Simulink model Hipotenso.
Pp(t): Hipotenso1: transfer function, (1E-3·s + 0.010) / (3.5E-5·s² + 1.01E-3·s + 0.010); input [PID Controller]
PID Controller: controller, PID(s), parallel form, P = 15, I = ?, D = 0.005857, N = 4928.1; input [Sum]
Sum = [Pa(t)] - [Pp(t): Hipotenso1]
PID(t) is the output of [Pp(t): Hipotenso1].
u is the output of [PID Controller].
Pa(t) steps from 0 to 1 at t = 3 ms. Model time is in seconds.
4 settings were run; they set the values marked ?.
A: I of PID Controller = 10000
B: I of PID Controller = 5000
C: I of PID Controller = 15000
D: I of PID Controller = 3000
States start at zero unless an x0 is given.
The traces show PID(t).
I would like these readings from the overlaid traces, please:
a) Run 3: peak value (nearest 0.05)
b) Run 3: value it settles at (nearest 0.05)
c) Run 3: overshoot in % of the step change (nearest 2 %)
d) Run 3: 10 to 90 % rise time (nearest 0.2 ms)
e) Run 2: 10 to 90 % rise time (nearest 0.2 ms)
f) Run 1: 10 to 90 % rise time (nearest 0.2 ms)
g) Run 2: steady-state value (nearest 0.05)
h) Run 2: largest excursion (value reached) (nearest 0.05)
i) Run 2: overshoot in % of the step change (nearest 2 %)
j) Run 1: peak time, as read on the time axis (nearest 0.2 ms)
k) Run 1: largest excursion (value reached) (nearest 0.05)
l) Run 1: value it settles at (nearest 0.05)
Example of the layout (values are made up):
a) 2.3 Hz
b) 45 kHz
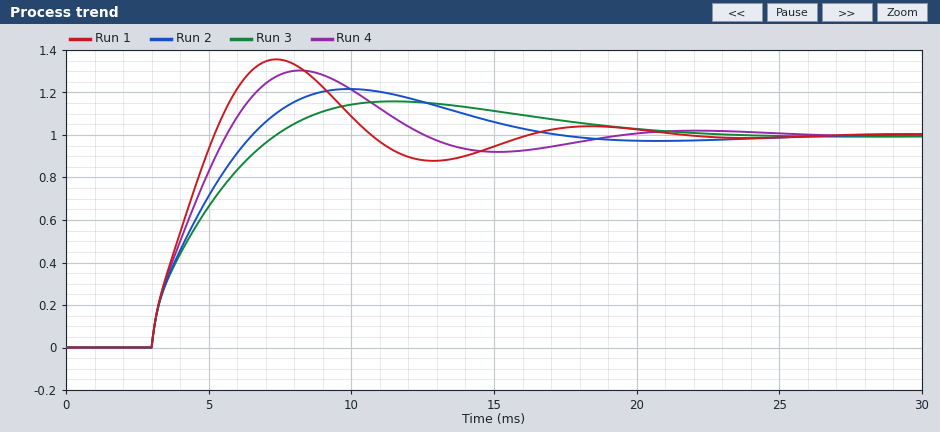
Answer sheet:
a) 1.15
b) 1.00
c) 16 %
d) 3.4 ms
e) 2.8 ms
f) 1.8 ms
g) 1.00
h) 1.20
i) 22 %
j) 7.4 ms
k) 1.35
l) 1.00
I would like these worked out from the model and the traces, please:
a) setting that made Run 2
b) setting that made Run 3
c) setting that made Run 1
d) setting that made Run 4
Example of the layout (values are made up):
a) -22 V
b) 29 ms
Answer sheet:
a) B
b) D
c) C
d) A
